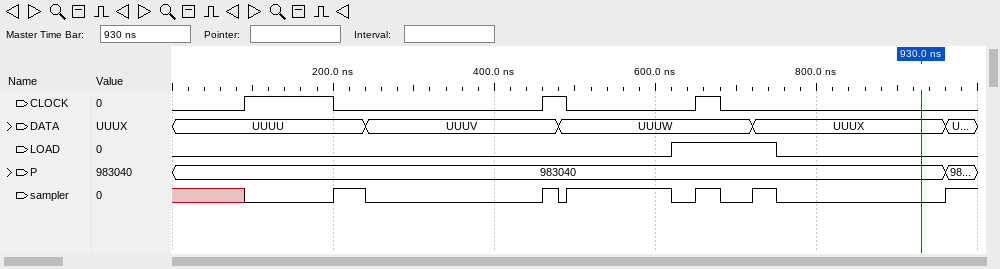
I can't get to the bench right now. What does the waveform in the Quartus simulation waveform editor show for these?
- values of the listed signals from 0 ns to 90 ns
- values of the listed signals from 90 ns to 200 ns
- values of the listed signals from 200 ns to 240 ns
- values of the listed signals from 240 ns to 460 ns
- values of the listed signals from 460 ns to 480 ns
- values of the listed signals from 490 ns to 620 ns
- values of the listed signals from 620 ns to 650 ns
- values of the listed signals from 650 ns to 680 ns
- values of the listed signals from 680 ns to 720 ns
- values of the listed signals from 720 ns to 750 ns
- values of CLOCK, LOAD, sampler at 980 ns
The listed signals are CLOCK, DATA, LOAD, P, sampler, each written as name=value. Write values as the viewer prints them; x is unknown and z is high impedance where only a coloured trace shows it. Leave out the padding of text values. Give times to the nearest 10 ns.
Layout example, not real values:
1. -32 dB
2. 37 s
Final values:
1. CLOCK=0, DATA=UUUU, LOAD=0, P=983040, sampler=x
2. CLOCK=1, DATA=UUUU, LOAD=0, P=983040, sampler=0
3. CLOCK=0, DATA=UUUU, LOAD=0, P=983040, sampler=1
4. CLOCK=0, DATA=UUUV, LOAD=0, P=983040, sampler=0
5. CLOCK=1, DATA=UUUV, LOAD=0, P=983040, sampler=1
6. CLOCK=0, DATA=UUUW, LOAD=0, P=983040, sampler=1
7. CLOCK=0, DATA=UUUW, LOAD=1, P=983040, sampler=0
8. CLOCK=1, DATA=UUUW, LOAD=1, P=983040, sampler=1
9. CLOCK=0, DATA=UUUW, LOAD=1, P=983040, sampler=0
10. CLOCK=0, DATA=UUUX, LOAD=1, P=983040, sampler=1
11. CLOCK=0, LOAD=0, sampler=1
